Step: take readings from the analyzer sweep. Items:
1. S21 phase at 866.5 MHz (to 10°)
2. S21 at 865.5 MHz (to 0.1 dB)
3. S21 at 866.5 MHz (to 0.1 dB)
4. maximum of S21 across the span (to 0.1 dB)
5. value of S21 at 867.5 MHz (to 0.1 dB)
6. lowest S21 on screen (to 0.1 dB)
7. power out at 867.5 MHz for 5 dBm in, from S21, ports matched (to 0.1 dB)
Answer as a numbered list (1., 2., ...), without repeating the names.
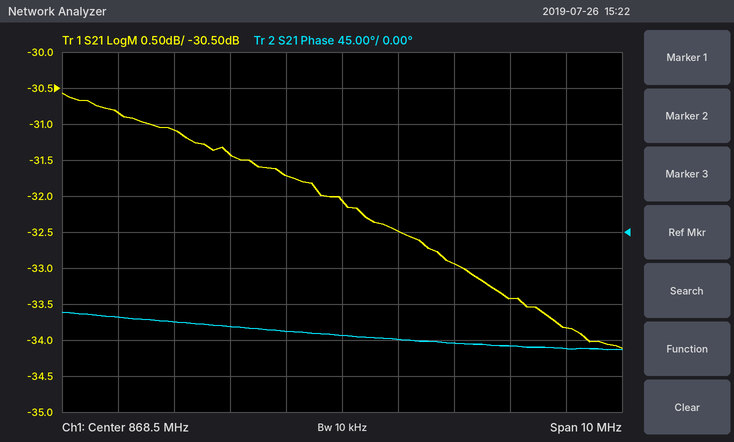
1. -120°
2. -31.1 dB
3. -31.4 dB
4. -30.6 dB
5. -31.7 dB
6. -34.1 dB
7. -26.7 dBm
